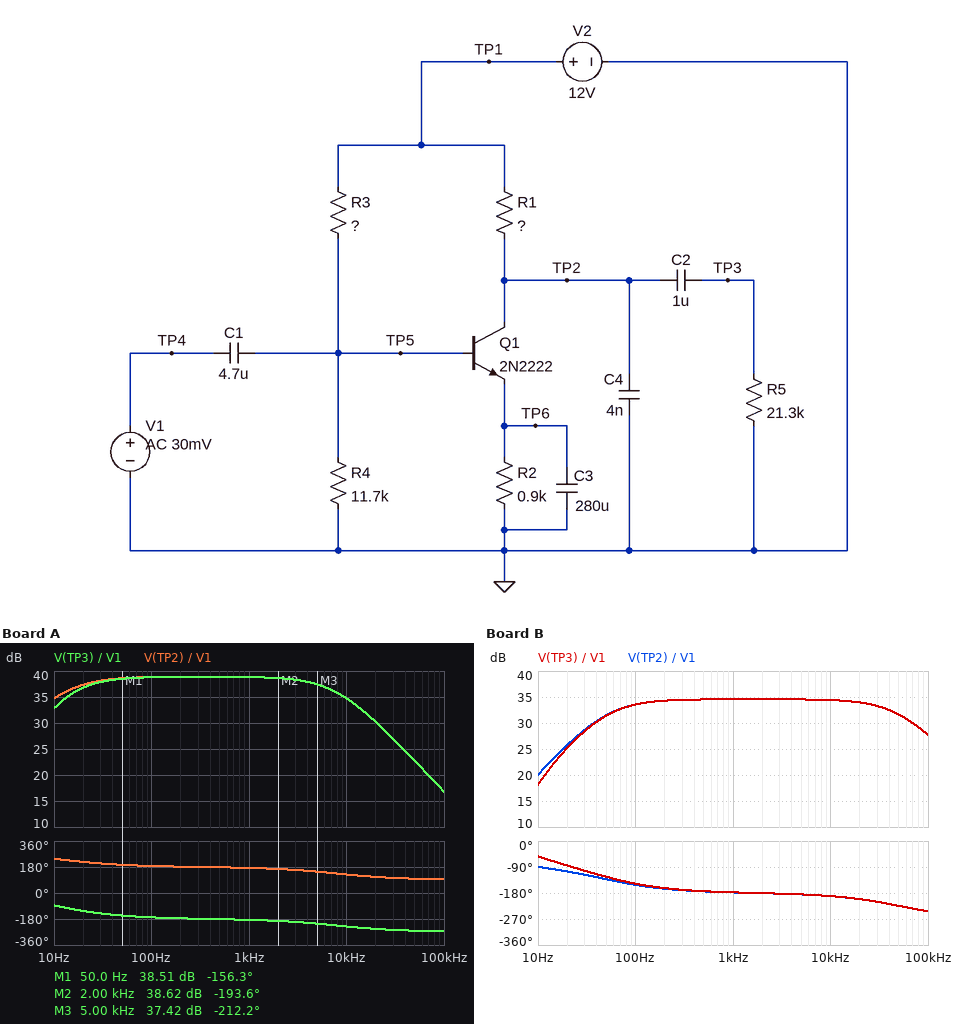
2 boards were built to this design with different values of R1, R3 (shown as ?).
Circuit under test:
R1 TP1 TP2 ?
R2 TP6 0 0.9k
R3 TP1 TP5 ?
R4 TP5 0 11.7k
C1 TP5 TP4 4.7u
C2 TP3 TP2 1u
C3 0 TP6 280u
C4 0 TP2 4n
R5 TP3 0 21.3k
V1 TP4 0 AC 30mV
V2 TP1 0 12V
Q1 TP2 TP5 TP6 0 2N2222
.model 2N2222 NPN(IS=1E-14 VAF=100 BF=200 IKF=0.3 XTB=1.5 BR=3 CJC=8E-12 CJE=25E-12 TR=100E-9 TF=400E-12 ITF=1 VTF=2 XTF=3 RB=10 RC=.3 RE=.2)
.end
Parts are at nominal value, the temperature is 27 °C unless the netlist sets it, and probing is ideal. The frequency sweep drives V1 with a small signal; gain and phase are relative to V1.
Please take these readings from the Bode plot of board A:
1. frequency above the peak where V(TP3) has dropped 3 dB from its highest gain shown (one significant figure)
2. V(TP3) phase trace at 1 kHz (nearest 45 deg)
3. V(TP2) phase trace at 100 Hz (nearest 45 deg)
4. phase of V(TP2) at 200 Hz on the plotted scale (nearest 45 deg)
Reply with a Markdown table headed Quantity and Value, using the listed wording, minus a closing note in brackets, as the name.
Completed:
| Quantity | Value |
|---|---|
| frequency above the peak where V(TP3) has dropped 3 dB from its highest gain shown | 8 kHz |
| V(TP3) phase trace at 1 kHz | -180 deg |
| V(TP2) phase trace at 100 Hz | 180 deg |
| phase of V(TP2) at 200 Hz on the plotted scale | 180 deg |
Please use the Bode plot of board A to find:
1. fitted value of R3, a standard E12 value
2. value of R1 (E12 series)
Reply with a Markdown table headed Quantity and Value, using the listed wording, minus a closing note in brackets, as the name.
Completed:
| Quantity | Value |
|---|---|
| fitted value of R3, a standard E12 value | 120 kΩ |
| value of R1 | 6.8 kΩ |
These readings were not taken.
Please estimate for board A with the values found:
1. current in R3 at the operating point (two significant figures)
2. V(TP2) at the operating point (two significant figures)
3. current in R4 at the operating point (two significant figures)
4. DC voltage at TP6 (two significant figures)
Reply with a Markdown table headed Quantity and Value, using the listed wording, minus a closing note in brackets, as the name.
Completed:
| Quantity | Value |
|---|---|
| current in R3 at the operating point | 91 µA |
| V(TP2) at the operating point | 8.9 V |
| current in R4 at the operating point | 89 µA |
| DC voltage at TP6 | 410 mV |
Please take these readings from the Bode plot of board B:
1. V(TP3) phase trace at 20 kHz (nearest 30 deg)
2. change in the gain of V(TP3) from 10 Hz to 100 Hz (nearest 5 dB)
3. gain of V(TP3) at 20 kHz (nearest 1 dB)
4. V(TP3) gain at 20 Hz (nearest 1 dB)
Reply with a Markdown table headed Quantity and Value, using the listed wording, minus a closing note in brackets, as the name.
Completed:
| Quantity | Value |
|---|---|
| V(TP3) phase trace at 20 kHz | -210 deg |
| change in the gain of V(TP3) from 10 Hz to 100 Hz | 15 dB |
| gain of V(TP3) at 20 kHz | 34 dB |
| V(TP3) gain at 20 Hz | 25 dB |
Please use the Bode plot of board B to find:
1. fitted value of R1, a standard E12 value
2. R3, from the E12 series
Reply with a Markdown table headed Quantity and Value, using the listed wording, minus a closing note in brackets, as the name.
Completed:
| Quantity | Value |
|---|---|
| fitted value of R1, a standard E12 value | 820 Ω |
| R3, from the E12 series | 47 kΩ |
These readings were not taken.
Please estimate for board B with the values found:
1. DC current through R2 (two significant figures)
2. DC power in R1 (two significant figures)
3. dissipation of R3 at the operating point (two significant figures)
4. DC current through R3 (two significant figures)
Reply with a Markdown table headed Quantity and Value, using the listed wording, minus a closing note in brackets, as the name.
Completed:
| Quantity | Value |
|---|---|
| DC current through R2 | 1.8 mA |
| DC power in R1 | 2.7 mW |
| dissipation of R3 at the operating point | 2.0 mW |
| DC current through R3 | 210 µA |
